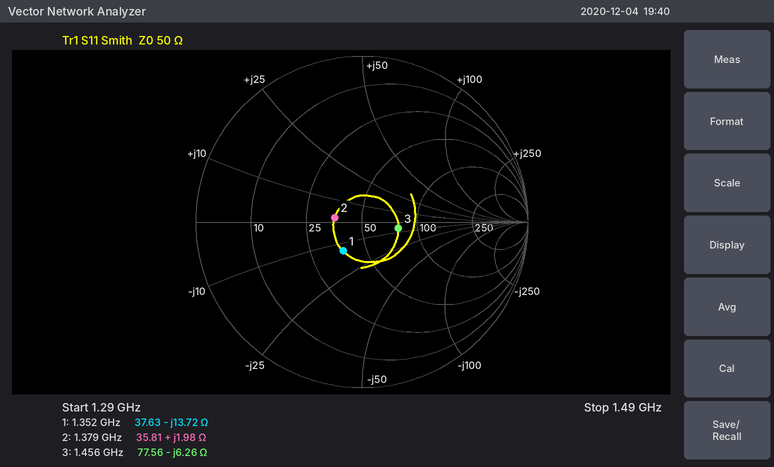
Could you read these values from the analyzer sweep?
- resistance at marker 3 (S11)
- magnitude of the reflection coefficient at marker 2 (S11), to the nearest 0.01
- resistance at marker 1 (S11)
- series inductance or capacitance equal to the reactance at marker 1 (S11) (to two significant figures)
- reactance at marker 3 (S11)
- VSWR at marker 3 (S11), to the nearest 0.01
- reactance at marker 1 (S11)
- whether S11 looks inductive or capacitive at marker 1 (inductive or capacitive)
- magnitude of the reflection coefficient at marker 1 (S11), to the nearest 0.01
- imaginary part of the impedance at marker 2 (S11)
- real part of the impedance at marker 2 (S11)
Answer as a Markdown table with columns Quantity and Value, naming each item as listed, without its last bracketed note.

| Quantity | Value |
|---|---|
| resistance at marker 3 | 77.56 Ω |
| magnitude of the reflection coefficient at marker 2 (S11), to the nearest 0.01 | 0.17 |
| resistance at marker 1 | 37.63 Ω |
| series inductance or capacitance equal to the reactance at marker 1 (S11) | 8.6 pF |
| reactance at marker 3 | -6.26 Ω |
| VSWR at marker 3 (S11), to the nearest 0.01 | 1.57 |
| reactance at marker 1 | -13.72 Ω |
| whether S11 looks inductive or capacitive at marker 1 | capacitive |
| magnitude of the reflection coefficient at marker 1 (S11), to the nearest 0.01 | 0.21 |
| imaginary part of the impedance at marker 2 | +1.98 Ω |
| real part of the impedance at marker 2 | 35.81 Ω |
